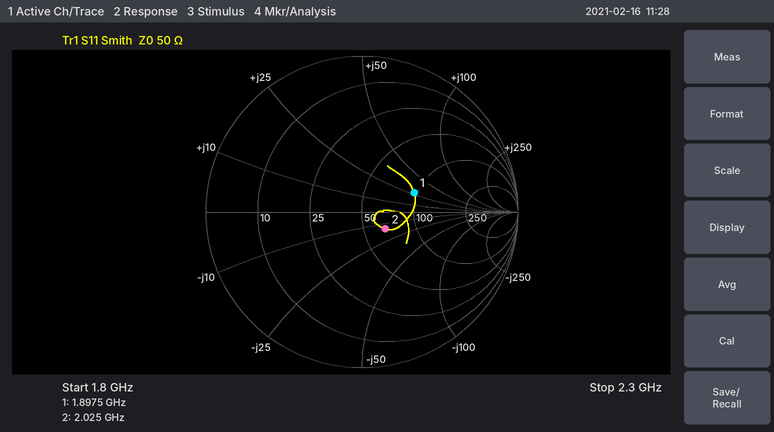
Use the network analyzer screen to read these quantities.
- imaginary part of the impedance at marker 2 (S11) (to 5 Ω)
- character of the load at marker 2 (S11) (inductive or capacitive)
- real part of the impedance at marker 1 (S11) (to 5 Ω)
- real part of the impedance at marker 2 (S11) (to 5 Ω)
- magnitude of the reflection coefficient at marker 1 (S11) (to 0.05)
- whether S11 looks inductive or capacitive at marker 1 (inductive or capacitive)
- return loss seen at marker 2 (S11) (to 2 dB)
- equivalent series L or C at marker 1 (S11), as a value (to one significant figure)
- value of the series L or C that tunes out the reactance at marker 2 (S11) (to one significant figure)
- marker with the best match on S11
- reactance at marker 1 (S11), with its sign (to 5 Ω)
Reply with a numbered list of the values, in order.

1. -15 Ω
2. capacitive
3. 95 Ω
4. 65 Ω
5. 0.35
6. inductive
7. 14 dB
8. 2 nH
9. 1 nH
10. marker 2
11. +25 Ω
